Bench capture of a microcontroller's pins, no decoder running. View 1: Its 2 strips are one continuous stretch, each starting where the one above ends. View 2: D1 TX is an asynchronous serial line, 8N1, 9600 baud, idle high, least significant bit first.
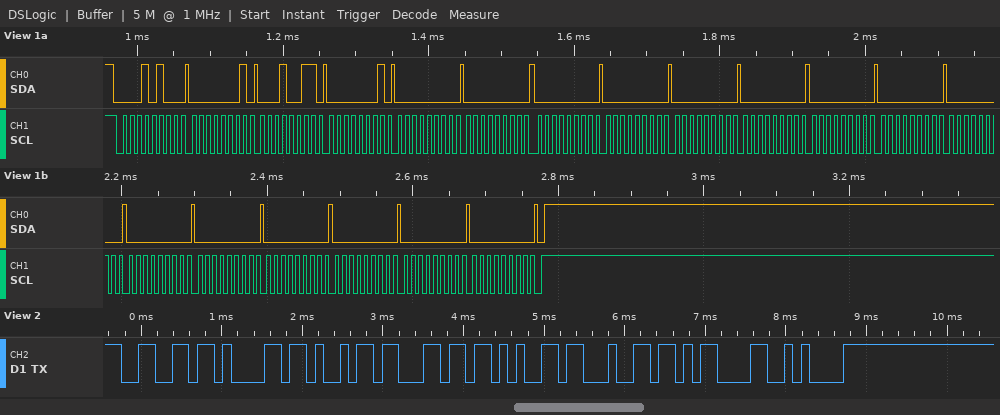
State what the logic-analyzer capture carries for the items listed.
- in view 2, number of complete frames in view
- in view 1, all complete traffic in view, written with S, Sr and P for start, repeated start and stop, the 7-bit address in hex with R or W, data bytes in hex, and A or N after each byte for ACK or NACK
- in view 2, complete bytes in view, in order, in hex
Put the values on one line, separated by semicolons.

8; S 0AW A 01 A 13 A 01 A 00 A 00 A 00 A 00 A 00 A 00 A 00 A 00 A 00 A 00 A 00 A 00 A 00 A 00 A 00 A P; 66 61 69 6C 65 64 0D 0A
